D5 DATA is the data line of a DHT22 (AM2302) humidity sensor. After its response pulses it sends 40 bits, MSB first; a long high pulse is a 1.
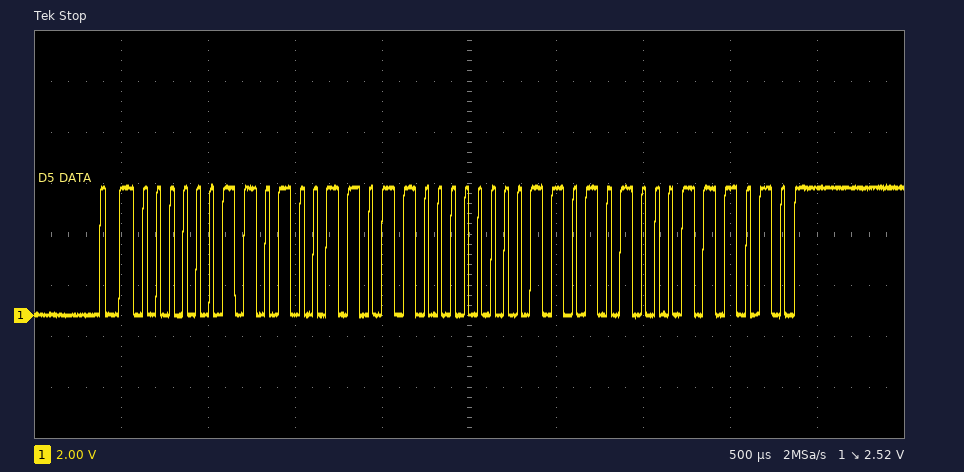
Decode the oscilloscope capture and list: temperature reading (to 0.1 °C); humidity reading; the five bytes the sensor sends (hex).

-10.6 °C
84.5 %
03 4D 80 6A 3A
